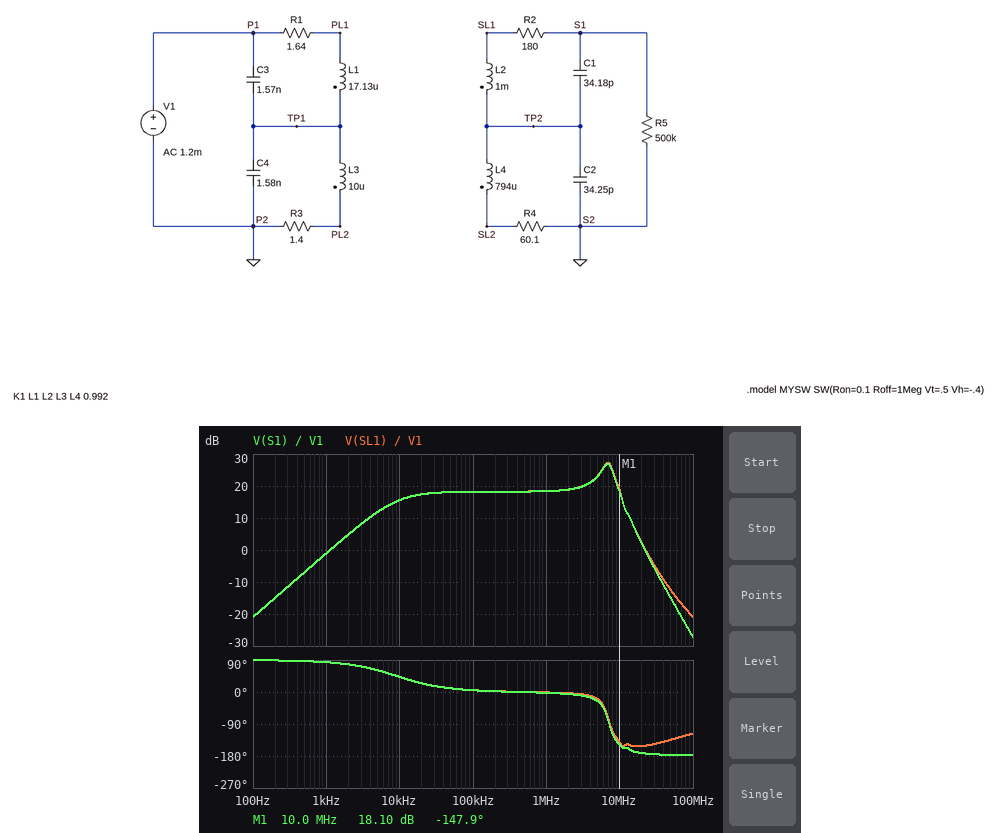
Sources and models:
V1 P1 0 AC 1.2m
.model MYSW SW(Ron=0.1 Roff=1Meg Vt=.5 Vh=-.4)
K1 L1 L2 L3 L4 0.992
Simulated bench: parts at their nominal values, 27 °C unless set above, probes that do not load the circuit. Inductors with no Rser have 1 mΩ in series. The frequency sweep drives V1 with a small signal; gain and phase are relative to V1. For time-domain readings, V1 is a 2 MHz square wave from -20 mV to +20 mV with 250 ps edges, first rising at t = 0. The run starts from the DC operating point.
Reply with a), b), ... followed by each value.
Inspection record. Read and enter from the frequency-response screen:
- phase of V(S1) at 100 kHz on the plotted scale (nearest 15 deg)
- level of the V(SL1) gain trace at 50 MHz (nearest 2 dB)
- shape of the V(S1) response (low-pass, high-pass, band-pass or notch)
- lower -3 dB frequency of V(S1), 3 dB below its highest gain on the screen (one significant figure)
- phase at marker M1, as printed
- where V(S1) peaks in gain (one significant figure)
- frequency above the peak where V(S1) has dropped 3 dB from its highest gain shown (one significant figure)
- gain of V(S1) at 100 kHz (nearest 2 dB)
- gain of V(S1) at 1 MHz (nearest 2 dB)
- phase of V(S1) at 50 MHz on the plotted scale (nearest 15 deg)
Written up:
a) 0 deg
b) -12 dB
c) band-pass
d) 5 MHz
e) -147.9 deg
f) 7 MHz
g) 8 MHz
h) 18 dB
i) 18 dB
j) -180 deg
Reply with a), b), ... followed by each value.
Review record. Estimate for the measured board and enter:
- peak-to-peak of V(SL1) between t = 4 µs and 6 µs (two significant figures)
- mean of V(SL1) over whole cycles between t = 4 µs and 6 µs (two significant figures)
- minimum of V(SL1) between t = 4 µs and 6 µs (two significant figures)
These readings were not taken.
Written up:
a) 730 mV
b) 120 mV
c) -240 mV
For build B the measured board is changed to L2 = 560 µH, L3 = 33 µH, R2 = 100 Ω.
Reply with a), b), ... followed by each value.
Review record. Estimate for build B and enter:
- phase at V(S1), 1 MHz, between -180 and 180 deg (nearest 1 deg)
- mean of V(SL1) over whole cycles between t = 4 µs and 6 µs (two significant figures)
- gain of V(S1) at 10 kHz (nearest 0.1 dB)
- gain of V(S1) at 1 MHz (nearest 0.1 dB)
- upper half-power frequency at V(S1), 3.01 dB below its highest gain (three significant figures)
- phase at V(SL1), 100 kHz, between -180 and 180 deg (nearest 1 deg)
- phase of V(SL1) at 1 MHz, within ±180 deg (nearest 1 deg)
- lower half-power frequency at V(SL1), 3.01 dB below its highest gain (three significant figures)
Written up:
a) -1 deg
b) 90 mV
c) 13.4 dB
d) 14.5 dB
e) 8.48 MHz
f) 3 deg
g) -1 deg
h) 7.08 MHz
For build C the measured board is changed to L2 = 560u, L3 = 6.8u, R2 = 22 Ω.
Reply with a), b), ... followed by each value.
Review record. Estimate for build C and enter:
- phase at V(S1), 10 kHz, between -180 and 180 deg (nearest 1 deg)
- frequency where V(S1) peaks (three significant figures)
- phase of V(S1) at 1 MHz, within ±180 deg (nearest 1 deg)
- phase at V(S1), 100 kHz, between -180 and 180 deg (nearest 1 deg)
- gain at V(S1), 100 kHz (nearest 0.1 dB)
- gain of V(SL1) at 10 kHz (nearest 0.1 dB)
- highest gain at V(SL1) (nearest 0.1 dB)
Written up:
a) 47 deg
b) 7.89 MHz
c) -1 deg
d) 6 deg
e) 17.6 dB
f) 14.4 dB
g) 29.8 dB
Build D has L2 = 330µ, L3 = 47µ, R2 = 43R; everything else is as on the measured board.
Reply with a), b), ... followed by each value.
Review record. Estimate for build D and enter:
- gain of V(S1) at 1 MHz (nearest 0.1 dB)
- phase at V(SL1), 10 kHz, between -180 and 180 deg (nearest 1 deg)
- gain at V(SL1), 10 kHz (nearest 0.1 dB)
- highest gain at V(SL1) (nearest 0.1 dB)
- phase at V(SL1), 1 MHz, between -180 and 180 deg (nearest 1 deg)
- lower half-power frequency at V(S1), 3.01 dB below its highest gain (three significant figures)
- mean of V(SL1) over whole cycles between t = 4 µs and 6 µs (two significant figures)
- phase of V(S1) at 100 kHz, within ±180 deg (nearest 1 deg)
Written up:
a) 12.6 dB
b) 22 deg
c) 11.8 dB
d) 24.8 dB
e) -1 deg
f) 7.14 MHz
g) 74 mV
h) 2 deg
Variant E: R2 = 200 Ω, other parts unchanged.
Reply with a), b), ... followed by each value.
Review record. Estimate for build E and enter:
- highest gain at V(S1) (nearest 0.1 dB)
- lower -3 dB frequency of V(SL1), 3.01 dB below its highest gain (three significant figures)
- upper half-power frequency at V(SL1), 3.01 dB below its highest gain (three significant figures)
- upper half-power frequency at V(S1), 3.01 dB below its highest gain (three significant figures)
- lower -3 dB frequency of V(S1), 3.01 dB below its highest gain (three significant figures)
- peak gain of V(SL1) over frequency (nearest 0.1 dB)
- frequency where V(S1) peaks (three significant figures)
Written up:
a) 26.6 dB
b) 5.35 MHz
c) 8.29 MHz
d) 8.20 MHz
e) 5.27 MHz
f) 26.9 dB
g) 6.88 MHz
